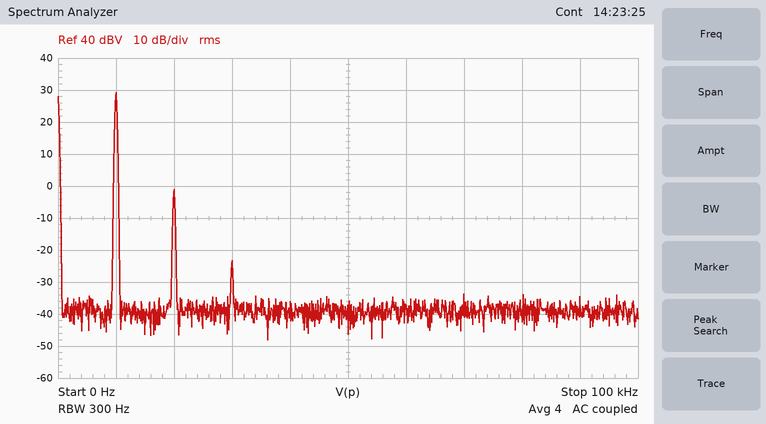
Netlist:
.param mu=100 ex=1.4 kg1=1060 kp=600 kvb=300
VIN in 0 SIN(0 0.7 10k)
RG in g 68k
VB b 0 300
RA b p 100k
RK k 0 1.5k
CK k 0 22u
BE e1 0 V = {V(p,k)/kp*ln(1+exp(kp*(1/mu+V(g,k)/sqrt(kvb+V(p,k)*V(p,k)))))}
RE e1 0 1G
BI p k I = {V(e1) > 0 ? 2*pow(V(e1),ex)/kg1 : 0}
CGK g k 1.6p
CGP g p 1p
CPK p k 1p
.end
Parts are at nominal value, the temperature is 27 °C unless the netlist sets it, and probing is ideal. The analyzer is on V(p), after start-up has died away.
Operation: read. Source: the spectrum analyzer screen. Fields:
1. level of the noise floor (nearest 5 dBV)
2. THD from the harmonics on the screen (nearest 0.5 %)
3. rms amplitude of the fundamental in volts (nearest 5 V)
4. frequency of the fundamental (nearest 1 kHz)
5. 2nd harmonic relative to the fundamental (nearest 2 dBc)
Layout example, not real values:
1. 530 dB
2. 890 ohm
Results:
1. -40 dBV
2. 3.0 %
3. 30 V
4. 10 kHz
5. -30 dBc
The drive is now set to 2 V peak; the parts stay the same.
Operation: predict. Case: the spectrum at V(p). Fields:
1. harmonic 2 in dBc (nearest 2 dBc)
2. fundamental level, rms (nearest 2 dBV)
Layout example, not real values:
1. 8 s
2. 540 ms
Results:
1. -20 dBc
2. 38 dBV
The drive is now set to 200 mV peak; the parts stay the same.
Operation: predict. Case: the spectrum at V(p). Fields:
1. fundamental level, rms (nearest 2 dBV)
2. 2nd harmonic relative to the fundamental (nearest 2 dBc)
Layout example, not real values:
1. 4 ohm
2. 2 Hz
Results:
1. 18 dBV
2. -42 dBc
